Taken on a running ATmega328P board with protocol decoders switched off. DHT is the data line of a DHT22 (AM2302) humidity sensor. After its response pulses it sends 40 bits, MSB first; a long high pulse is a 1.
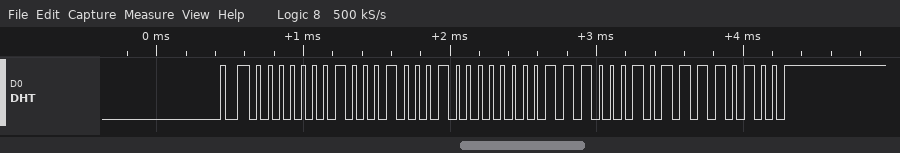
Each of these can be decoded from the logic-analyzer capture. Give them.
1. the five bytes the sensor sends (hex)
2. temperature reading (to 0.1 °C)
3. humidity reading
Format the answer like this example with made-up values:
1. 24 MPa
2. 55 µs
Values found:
1. 01 11 00 E2 F4
2. 22.6 °C
3. 27.3 %
